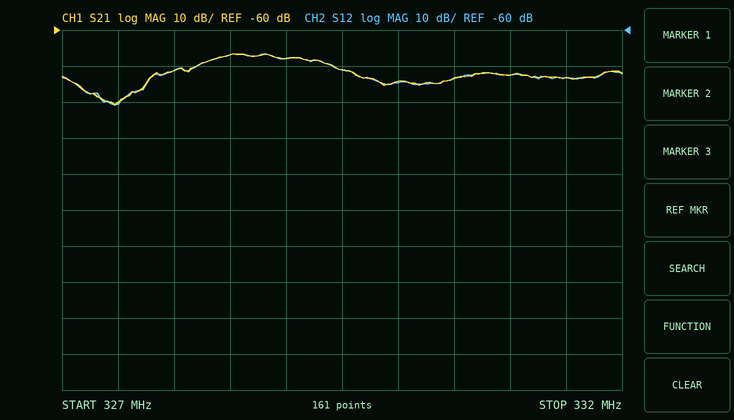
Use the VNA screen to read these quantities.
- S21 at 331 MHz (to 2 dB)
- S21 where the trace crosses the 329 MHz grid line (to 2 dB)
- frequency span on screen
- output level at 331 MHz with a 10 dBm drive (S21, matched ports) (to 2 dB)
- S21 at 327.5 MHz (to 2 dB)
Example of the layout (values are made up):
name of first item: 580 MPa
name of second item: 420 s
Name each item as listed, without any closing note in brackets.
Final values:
S21 at 331 MHz: -72 dB
S21 where the trace crosses the 329 MHz grid line: -68 dB
frequency span on screen: 5 MHz
output level at 331 MHz with a 10 dBm drive (S21, matched ports): -62 dBm
S21 at 327.5 MHz: -80 dB
